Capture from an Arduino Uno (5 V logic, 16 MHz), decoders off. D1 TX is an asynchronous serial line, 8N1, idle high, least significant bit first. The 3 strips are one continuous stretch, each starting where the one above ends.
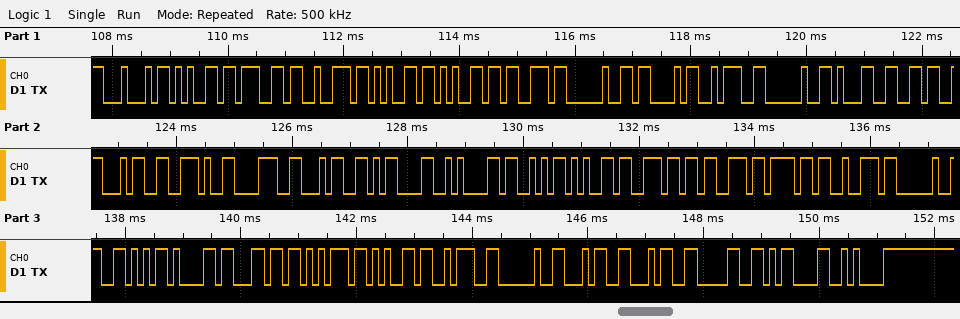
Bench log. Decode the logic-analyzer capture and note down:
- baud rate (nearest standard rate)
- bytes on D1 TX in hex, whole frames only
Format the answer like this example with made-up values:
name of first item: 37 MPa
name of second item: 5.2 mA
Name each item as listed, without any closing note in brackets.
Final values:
baud rate: 9600 baud
bytes on D1 TX in hex, whole frames only: 0x44 0x65 0x67 0x72 0x65 0x65 0x73 0x20 0x43 0x3A 0x20 0x31 0x36 0x34 0x2E 0x38 0x34 0x0D 0x0A 0x53 0x65 0x6E 0x73 0x6F 0x72 0x20 0x56 0x61 0x6C 0x75 0x65 0x3A 0x20 0x34 0x34 0x30 0x0D 0x0A
